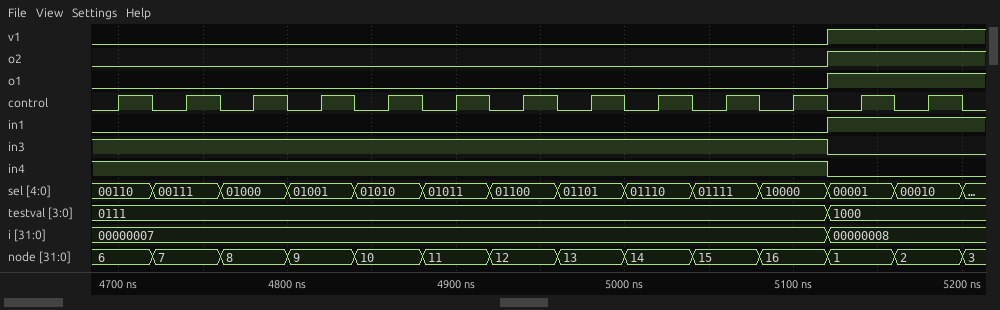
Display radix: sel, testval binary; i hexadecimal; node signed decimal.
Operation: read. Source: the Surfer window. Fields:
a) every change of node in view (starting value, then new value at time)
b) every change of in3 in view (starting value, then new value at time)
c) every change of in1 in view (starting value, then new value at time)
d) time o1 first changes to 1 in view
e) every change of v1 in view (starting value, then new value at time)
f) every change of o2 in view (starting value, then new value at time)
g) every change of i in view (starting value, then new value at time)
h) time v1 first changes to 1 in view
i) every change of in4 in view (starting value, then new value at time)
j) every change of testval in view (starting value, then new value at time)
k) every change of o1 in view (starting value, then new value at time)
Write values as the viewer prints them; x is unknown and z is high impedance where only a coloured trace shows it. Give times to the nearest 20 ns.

6, 7 at 4720 ns, 8 at 4760 ns, 9 at 4800 ns, 10 at 4840 ns, 11 at 4880 ns, 12 at 4920 ns, 13 at 4960 ns, 14 at 5000 ns, 15 at 5040 ns, 16 at 5080 ns, 1 at 5120 ns, 2 at 5160 ns, 3 at 5200 ns
1, 0 at 5120 ns
0, 1 at 5120 ns
5120 ns
0, 1 at 5120 ns
0, 1 at 5120 ns
00000007, 00000008 at 5120 ns
5120 ns
1, 0 at 5120 ns
0111, 1000 at 5120 ns
0, 1 at 5120 ns
